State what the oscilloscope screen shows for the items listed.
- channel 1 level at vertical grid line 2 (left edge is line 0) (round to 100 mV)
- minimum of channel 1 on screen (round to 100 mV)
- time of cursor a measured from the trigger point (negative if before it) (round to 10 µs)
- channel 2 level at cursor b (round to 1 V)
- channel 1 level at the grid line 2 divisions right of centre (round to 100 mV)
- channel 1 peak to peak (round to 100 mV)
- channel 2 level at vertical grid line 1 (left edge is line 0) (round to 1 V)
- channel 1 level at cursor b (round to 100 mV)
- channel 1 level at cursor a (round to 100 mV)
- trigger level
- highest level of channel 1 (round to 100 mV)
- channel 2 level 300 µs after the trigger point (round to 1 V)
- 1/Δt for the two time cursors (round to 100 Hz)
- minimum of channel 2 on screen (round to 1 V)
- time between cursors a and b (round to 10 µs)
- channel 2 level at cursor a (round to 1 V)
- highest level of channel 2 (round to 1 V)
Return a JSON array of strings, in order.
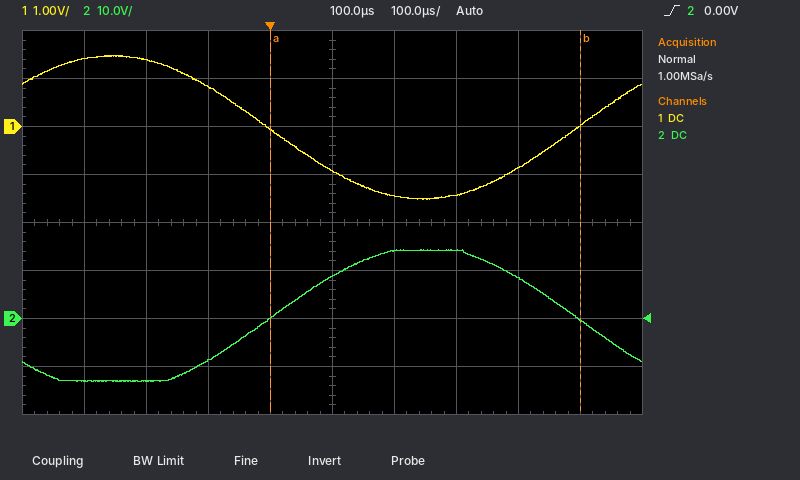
["1.4 V", "-1.5 V", "0 µs", "0 V", "-1.4 V", "3.0 V", "-13 V", "0.0 V", "-100 mV", "0.00 V", "1.5 V", "14 V", "2.0 kHz", "-13 V", "500 µs", "0 V", "14 V"]
